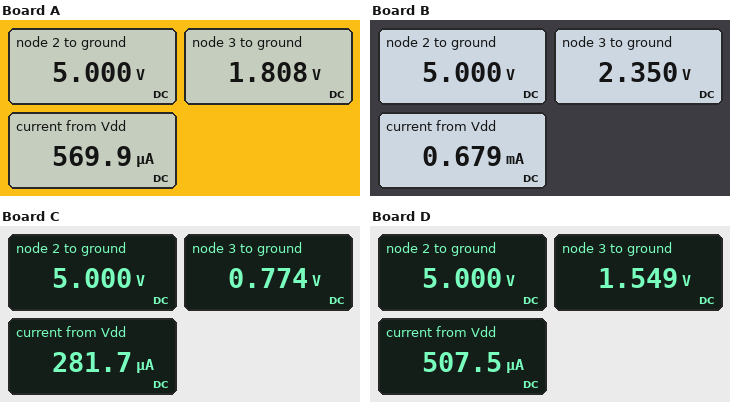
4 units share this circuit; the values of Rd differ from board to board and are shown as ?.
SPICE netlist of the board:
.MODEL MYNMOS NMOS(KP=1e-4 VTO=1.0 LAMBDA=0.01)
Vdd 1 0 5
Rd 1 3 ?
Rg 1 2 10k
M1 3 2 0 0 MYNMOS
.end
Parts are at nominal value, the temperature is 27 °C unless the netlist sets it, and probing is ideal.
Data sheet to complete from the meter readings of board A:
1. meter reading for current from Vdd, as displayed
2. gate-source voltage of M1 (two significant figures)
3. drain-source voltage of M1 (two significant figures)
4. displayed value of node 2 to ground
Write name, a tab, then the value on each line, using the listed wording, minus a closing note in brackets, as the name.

meter reading for current from Vdd, as displayed	569.9 µA
gate-source voltage of M1	5.0 V
drain-source voltage of M1	1.8 V
displayed value of node 2 to ground	5.000 V
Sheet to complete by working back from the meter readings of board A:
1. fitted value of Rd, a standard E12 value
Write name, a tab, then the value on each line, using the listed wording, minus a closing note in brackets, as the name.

fitted value of Rd, a standard E12 value	5.6 kΩ
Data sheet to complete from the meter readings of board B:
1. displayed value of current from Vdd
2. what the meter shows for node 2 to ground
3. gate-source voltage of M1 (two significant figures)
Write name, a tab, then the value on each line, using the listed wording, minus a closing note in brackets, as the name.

displayed value of current from Vdd	0.679 mA
what the meter shows for node 2 to ground	5.000 V
gate-source voltage of M1	5.0 V
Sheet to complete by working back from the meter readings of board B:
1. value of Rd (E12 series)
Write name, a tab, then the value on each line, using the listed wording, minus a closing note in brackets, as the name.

value of Rd	3.9 kΩ
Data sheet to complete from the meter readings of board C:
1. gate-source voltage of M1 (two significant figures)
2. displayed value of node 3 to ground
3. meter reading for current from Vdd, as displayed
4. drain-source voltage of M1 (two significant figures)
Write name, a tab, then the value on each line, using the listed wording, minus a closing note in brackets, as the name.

gate-source voltage of M1	5.0 V
displayed value of node 3 to ground	0.774 V
meter reading for current from Vdd, as displayed	281.7 µA
drain-source voltage of M1	770 mV
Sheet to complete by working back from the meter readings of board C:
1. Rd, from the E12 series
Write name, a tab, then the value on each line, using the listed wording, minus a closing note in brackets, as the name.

Rd, from the E12 series	15 kΩ
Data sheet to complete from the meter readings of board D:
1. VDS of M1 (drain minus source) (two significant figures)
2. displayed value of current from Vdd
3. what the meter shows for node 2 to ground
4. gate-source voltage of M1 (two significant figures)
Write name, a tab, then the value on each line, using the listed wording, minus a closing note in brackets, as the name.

VDS of M1 (drain minus source)	1.5 V
displayed value of current from Vdd	507.5 µA
what the meter shows for node 2 to ground	5.000 V
gate-source voltage of M1	5.0 V
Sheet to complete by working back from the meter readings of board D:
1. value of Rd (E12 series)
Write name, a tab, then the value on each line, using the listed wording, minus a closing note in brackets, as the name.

value of Rd	6.8 kΩ
